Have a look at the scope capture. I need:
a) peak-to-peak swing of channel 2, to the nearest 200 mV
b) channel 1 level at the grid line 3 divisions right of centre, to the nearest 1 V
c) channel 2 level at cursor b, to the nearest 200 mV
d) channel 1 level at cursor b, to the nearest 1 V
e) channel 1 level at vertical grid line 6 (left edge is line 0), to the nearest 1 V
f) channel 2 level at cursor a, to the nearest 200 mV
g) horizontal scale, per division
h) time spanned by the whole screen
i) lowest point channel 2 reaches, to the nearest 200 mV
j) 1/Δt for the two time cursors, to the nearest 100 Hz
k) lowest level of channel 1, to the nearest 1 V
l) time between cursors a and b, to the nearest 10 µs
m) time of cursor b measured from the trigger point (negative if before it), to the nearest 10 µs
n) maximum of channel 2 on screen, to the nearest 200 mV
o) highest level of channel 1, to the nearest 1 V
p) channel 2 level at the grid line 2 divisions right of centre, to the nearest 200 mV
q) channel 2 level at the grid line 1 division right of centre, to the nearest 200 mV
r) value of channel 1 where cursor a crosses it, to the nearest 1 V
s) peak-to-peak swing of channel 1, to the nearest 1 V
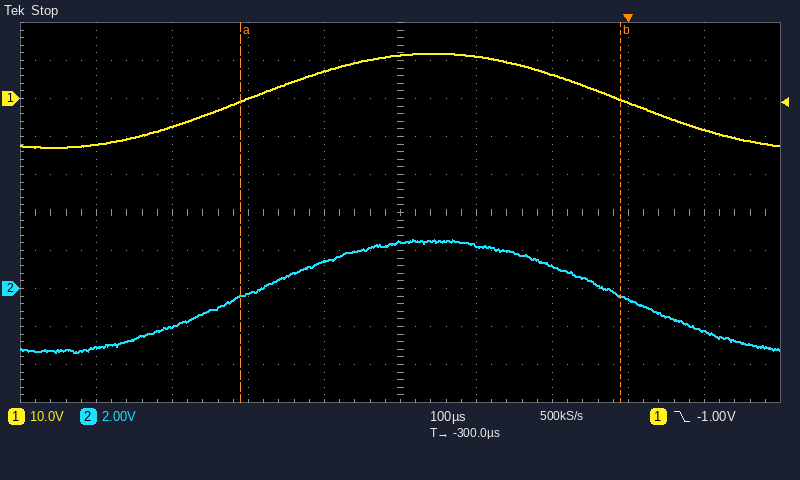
6.0 V
-1 V
-400 mV
0 V
11 V
-400 mV
100 µs
1 ms
-3.4 V
2.0 kHz
-13 V
500 µs
-10 µs
2.6 V
12 V
1.2 V
2.2 V
-1 V
25 V
